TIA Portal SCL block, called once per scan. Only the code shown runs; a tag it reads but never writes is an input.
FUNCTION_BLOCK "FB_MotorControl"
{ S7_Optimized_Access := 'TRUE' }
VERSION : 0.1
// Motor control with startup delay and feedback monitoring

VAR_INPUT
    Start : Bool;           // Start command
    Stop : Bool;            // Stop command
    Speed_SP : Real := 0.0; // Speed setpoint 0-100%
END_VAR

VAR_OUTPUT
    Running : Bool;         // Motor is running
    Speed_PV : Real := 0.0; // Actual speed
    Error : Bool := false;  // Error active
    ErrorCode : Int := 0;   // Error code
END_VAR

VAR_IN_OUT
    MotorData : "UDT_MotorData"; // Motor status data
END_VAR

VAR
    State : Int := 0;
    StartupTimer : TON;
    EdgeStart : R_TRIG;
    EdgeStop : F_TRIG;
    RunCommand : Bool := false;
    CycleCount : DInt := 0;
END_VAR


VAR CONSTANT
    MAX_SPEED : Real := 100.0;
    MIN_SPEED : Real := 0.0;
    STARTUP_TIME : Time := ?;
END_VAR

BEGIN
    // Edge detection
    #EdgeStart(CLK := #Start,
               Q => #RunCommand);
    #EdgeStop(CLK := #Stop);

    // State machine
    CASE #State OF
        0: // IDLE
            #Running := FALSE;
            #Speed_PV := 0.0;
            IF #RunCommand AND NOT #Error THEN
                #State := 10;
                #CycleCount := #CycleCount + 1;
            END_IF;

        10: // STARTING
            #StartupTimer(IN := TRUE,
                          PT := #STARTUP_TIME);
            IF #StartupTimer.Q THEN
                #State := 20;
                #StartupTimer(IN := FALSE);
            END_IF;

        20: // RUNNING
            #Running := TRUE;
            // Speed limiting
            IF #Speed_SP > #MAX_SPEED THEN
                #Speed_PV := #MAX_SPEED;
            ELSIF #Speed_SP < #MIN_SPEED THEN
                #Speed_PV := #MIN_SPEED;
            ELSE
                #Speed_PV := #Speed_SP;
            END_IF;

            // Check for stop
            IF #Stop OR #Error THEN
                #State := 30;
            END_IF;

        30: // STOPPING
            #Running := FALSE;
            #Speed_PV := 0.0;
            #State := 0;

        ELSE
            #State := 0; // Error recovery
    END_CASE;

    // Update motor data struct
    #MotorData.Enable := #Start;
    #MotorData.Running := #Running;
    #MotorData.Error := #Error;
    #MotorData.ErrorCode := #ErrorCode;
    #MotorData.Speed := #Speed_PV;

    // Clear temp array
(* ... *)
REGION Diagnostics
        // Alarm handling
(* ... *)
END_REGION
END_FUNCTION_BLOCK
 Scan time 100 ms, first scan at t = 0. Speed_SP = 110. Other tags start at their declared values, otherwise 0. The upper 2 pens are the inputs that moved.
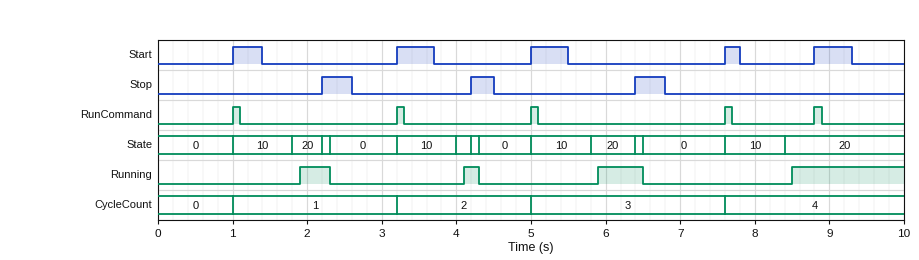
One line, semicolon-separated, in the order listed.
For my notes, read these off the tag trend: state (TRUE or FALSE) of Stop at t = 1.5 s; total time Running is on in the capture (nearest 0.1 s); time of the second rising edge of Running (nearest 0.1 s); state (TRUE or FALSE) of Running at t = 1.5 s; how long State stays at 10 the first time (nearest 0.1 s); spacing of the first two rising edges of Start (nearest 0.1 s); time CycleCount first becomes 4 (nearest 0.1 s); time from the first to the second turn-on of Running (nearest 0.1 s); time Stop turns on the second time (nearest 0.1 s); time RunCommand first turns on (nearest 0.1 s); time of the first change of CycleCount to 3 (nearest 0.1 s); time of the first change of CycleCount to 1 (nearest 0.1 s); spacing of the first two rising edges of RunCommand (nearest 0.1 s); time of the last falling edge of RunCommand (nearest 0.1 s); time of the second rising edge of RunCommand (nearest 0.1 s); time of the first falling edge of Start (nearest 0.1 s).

FALSE; 2.7 s; 4.1 s; FALSE; 0.8 s; 2.2 s; 7.6 s; 2.2 s; 4.2 s; 1.0 s; 5.0 s; 1.0 s; 2.2 s; 8.9 s; 3.2 s; 1.4 s
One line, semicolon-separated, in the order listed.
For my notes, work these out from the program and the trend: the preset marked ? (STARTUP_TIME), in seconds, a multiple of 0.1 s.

0.7 s
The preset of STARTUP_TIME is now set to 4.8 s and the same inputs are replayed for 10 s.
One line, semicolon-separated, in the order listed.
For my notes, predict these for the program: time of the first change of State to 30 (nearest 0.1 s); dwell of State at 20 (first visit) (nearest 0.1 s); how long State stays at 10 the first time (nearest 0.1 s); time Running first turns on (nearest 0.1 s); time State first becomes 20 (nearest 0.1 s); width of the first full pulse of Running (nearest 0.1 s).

6.4 s; 0.5 s; 4.9 s; 6.0 s; 5.9 s; 0.5 s
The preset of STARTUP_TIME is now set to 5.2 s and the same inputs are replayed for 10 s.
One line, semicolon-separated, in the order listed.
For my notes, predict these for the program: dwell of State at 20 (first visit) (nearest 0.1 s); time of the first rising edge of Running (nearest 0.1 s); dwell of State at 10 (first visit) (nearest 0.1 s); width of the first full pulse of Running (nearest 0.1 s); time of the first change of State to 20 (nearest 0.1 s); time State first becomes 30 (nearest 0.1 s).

0.1 s; 6.4 s; 5.3 s; 0.1 s; 6.3 s; 6.4 s
